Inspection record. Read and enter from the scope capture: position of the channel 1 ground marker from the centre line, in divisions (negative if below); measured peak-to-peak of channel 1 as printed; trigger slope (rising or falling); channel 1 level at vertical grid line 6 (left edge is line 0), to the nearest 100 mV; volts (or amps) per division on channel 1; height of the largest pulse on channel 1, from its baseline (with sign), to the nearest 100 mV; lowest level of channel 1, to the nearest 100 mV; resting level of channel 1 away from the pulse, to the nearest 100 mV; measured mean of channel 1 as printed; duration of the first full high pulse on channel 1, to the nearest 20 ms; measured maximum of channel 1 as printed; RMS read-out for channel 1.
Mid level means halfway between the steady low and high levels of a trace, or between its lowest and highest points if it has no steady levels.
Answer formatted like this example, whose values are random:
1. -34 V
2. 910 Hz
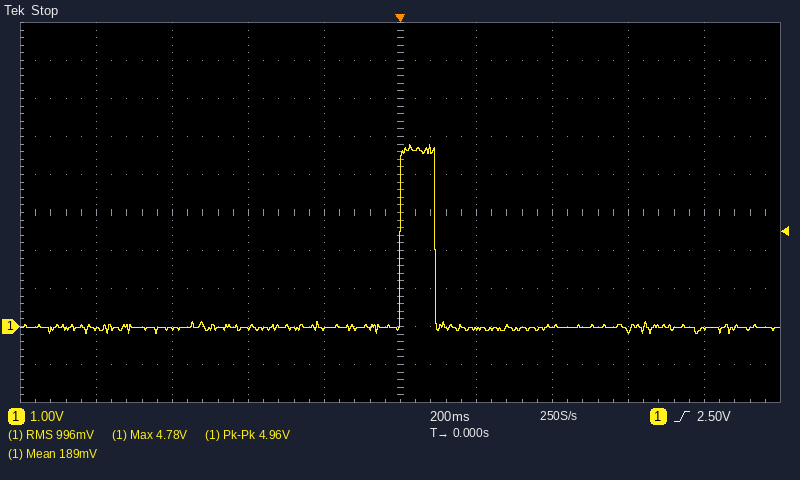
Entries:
1. -3.0 div
2. 4.96 V
3. rising
4. -100 mV
5. 1 V
6. +4.8 V
7. -200 mV
8. 0.0 V
9. 189 mV
10. 100 ms
11. 4.78 V
12. 996 mV
